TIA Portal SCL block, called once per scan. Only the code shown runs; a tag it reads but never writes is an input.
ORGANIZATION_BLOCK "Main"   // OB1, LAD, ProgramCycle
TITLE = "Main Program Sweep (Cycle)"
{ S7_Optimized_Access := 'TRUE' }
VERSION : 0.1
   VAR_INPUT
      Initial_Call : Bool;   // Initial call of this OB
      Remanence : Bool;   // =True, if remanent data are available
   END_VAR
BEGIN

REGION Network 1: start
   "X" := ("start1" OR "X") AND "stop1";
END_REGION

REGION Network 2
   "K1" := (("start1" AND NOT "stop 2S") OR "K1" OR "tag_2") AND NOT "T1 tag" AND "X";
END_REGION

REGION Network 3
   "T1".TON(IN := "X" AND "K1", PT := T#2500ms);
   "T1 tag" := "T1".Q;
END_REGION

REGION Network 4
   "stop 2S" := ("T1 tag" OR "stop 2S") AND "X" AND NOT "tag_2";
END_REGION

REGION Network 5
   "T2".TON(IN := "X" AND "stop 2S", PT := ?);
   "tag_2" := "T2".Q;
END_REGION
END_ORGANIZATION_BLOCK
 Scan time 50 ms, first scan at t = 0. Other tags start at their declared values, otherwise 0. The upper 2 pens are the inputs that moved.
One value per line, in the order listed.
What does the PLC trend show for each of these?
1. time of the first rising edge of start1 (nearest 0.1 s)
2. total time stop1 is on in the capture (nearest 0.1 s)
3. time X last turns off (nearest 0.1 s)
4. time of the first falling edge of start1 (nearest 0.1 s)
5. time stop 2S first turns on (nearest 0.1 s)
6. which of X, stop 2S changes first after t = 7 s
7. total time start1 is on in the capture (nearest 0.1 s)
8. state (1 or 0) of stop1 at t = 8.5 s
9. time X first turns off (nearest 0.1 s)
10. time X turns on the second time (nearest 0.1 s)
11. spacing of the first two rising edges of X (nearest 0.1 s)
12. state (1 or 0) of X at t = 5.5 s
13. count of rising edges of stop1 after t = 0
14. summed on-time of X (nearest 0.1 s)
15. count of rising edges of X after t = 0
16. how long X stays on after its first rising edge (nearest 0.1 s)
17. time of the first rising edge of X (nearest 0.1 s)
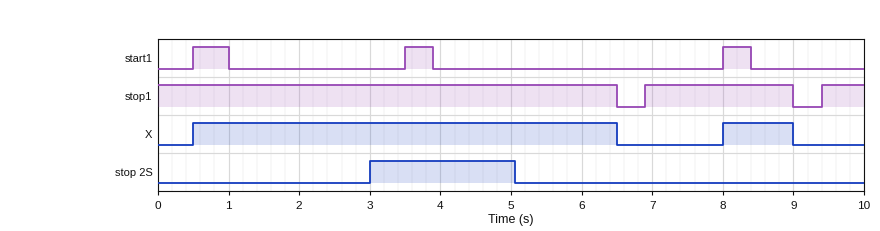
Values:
0.5 s
9.2 s
9.0 s
1.0 s
3.0 s
X
1.3 s
1
6.5 s
8.0 s
7.5 s
1
2
7.0 s
2
6.0 s
0.5 s
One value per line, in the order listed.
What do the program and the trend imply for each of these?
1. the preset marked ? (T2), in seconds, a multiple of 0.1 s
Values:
2.0 s
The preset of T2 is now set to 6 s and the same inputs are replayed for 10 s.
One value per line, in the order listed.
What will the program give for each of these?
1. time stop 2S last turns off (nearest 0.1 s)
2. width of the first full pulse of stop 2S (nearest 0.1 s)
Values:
6.5 s
3.5 s
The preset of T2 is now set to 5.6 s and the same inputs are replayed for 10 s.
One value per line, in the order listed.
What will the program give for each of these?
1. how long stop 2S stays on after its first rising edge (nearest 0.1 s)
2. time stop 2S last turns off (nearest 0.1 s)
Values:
3.5 s
6.5 s
